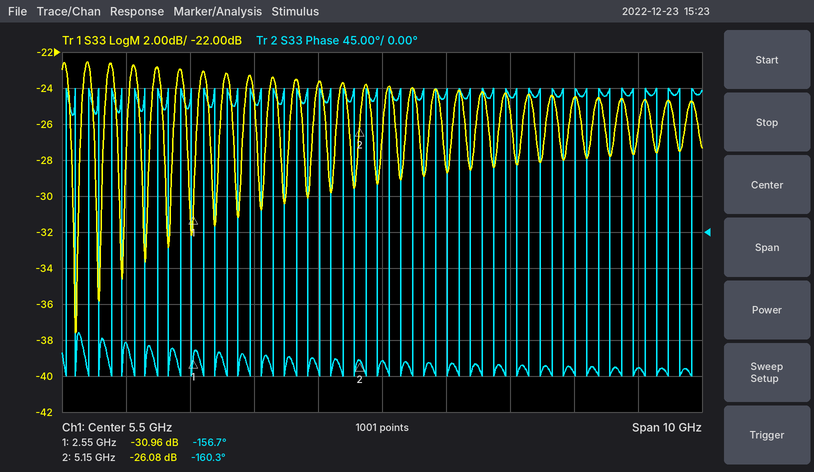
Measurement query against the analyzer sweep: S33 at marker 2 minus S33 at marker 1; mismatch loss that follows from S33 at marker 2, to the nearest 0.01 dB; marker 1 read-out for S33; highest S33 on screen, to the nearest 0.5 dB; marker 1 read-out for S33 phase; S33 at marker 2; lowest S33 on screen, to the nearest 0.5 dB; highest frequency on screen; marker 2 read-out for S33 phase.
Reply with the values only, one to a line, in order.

4.88 dB
0.01 dB
-30.96 dB
-22.5 dB
-156.7°
-26.08 dB
-37.5 dB
10.5 GHz
-160.3°
